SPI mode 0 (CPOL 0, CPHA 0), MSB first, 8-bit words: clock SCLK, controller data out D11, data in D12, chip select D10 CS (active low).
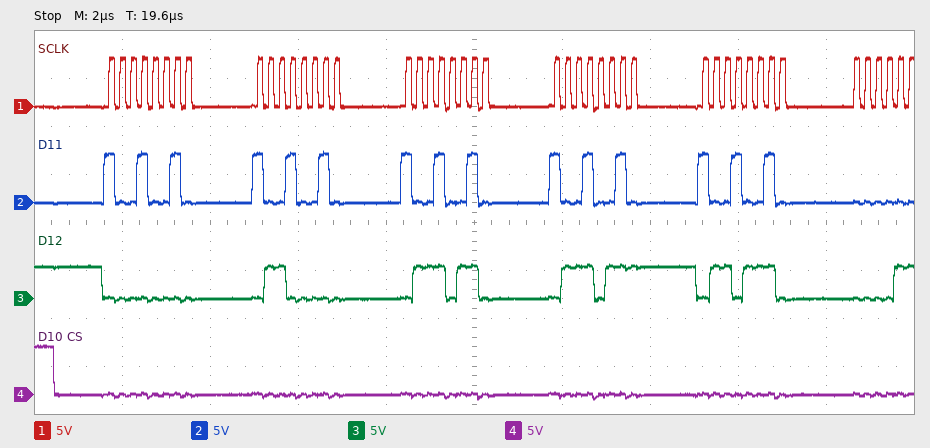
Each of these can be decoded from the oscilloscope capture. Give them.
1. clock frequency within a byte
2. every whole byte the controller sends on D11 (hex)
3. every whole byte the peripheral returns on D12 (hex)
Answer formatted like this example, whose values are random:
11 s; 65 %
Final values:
4 MHz; 92 92 92 92 92; 00 60 76 77 6E
